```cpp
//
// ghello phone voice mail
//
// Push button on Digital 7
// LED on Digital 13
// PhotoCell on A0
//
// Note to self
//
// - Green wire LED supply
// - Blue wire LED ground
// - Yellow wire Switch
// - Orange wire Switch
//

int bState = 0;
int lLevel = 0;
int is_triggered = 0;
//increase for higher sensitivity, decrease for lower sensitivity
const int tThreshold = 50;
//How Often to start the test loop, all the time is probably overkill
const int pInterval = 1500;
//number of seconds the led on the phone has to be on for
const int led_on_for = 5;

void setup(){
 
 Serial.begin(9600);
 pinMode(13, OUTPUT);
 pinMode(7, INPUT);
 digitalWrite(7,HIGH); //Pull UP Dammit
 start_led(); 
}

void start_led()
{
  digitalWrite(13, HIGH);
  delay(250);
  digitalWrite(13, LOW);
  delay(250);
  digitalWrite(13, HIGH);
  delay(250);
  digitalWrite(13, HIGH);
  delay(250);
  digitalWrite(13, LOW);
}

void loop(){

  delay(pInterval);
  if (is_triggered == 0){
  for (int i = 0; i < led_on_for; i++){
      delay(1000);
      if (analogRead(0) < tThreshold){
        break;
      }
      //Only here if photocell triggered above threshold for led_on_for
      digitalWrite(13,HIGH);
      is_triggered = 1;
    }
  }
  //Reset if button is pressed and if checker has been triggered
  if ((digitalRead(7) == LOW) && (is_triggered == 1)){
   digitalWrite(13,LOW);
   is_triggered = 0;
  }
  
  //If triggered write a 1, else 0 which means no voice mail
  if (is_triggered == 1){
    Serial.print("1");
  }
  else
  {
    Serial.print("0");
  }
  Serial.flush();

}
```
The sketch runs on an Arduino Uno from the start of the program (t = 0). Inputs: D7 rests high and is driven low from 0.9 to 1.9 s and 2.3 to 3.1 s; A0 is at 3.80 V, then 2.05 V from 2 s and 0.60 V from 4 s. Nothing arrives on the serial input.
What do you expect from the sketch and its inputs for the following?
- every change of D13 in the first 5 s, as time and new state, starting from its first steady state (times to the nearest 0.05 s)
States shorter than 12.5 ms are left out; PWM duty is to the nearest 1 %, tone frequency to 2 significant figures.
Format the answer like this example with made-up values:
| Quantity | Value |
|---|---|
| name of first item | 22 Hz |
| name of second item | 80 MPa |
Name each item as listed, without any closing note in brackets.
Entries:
| Quantity | Value |
|---|---|
| every change of D13 in the first 5 s, as time and new state, starting from its first steady state | 0 s high; 0.25 s low; 0.5 s high; 1 s low; 3.5 s high |
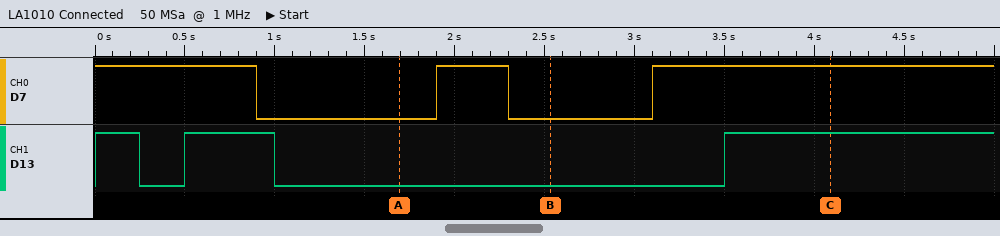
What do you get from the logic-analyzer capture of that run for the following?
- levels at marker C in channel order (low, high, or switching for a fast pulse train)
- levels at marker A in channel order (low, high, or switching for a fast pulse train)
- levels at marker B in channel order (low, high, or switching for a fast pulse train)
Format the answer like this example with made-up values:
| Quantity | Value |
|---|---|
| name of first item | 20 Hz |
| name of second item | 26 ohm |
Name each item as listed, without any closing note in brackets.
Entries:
| Quantity | Value |
|---|---|
| levels at marker C in channel order | D7 high, D13 high |
| levels at marker A in channel order | D7 low, D13 low |
| levels at marker B in channel order | D7 low, D13 low |
